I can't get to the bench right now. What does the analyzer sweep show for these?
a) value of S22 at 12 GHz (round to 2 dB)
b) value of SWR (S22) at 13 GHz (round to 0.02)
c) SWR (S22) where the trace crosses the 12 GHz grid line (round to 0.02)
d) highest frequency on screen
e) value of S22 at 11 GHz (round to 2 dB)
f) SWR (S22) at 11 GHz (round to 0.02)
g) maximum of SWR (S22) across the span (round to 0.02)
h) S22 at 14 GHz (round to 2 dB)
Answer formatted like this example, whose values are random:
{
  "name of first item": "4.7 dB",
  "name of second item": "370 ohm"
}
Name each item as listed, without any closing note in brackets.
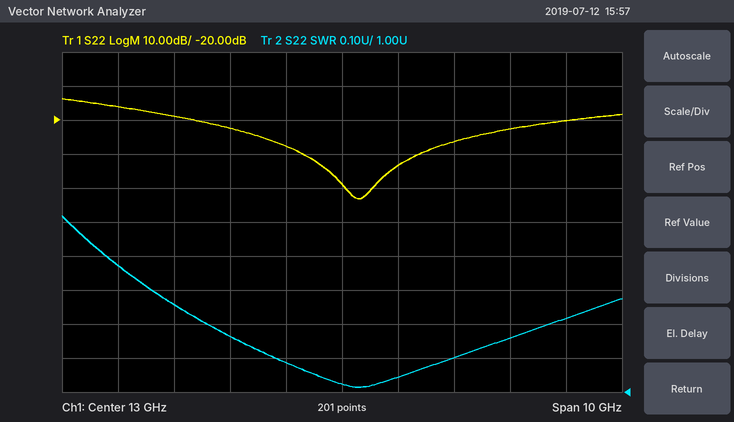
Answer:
{
  "value of S22 at 12 GHz": "-28 dB",
  "value of SWR (S22) at 13 GHz": "1.02",
  "SWR (S22) where the trace crosses the 12 GHz grid line": "1.08",
  "highest frequency on screen": "18 GHz",
  "value of S22 at 11 GHz": "-22 dB",
  "SWR (S22) at 11 GHz": "1.16",
  "maximum of SWR (S22) across the span": "1.52",
  "S22 at 14 GHz": "-34 dB"
}
